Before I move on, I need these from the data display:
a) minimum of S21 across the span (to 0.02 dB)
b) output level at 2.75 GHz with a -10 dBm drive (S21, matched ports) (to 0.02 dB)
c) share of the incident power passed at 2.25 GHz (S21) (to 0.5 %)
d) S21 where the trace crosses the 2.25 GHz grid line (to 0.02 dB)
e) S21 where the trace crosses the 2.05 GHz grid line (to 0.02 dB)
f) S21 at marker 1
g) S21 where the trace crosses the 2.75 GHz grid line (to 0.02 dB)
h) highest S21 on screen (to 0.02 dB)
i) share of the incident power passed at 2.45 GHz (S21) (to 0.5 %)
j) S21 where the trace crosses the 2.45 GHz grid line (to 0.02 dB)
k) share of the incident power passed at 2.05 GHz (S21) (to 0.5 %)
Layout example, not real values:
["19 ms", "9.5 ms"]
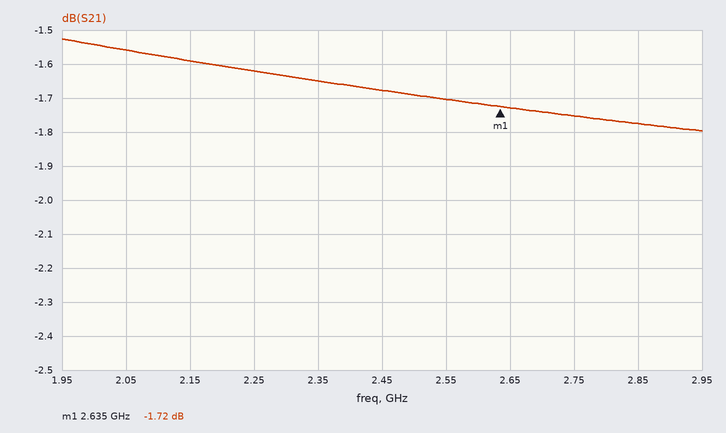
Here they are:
["-1.80 dB", "-11.76 dBm", "69.0 %", "-1.62 dB", "-1.56 dB", "-1.72 dB", "-1.76 dB", "-1.52 dB", "68.0 %", "-1.68 dB", "70.0 %"]
